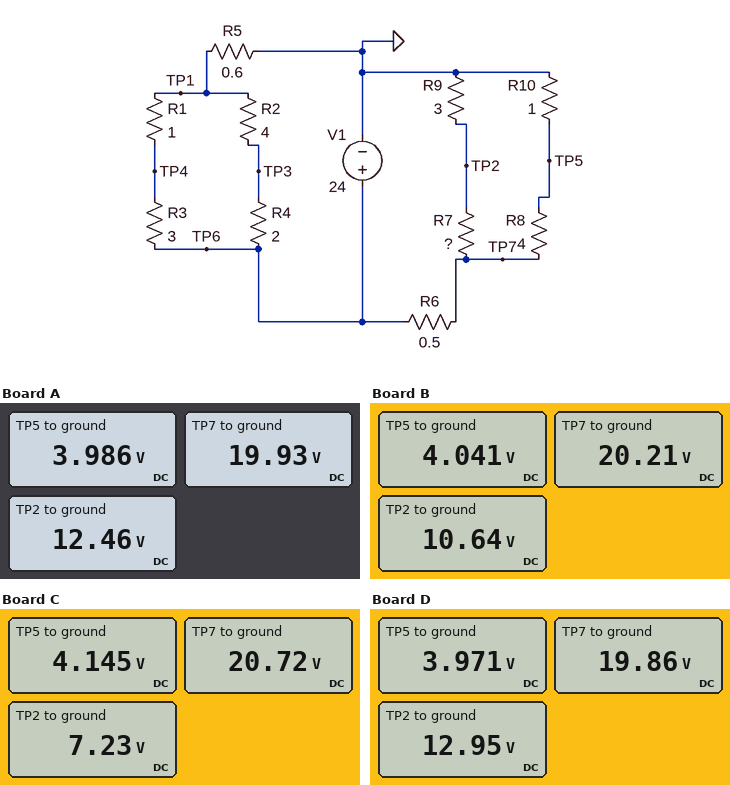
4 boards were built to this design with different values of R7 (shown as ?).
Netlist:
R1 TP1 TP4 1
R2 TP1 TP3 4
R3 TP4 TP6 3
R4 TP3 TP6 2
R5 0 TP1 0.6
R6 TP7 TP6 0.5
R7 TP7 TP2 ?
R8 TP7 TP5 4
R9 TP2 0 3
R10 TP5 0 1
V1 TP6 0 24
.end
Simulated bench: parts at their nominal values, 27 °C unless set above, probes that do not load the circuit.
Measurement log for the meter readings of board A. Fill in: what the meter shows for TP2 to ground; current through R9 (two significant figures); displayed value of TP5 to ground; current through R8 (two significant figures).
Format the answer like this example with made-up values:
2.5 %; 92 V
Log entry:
12.46 V; 4.2 A; 3.986 V; 4.0 A
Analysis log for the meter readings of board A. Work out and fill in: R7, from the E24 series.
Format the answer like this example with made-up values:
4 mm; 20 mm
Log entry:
1.8 Ω
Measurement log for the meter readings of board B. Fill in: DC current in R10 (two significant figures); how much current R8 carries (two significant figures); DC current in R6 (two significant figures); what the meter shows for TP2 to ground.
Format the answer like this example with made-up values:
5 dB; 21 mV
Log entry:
4.0 A; 4.0 A; 7.6 A; 10.64 V
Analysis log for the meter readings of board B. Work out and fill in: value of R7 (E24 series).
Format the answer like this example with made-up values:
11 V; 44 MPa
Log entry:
2.7 Ω
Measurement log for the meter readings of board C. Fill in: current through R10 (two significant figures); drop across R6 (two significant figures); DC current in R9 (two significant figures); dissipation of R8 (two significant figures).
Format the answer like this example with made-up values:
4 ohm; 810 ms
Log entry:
4.1 A; 3.3 V; 2.4 A; 69 W
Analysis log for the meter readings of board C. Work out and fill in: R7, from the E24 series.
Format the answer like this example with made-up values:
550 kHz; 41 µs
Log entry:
5.6 Ω
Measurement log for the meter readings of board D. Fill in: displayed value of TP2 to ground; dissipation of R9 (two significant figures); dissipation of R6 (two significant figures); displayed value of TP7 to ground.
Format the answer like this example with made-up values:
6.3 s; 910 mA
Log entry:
12.95 V; 56 W; 34 W; 19.86 V
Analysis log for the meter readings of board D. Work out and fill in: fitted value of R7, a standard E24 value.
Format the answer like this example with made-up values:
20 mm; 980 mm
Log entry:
1.6 Ω
